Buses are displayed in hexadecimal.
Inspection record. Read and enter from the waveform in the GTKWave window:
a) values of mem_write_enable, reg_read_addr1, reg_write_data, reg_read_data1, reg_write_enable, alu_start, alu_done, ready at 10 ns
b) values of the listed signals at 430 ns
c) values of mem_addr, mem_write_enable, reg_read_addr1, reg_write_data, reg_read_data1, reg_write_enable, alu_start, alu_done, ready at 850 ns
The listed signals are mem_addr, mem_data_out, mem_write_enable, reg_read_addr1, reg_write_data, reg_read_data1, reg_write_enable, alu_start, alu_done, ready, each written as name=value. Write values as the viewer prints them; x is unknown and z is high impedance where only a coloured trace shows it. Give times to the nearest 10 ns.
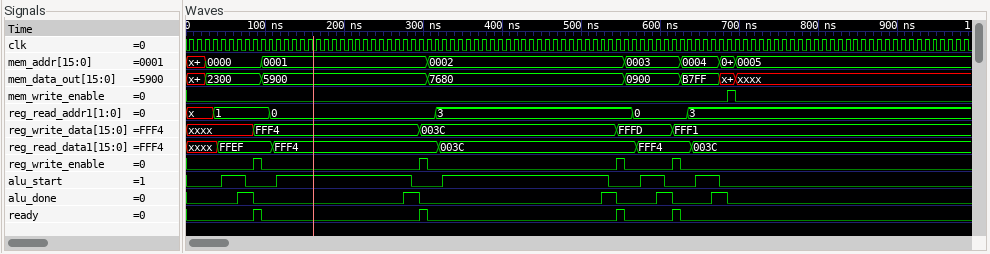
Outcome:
mem_write_enable=0, reg_read_addr1=x, reg_write_data=xxxx, reg_read_data1=xxxx, reg_write_enable=0, alu_start=0, alu_done=0, ready=0
mem_addr=0002, mem_data_out=7680, mem_write_enable=0, reg_read_addr1=3, reg_write_data=003C, reg_read_data1=003C, reg_write_enable=0, alu_start=1, alu_done=0, ready=0
mem_addr=0005, mem_write_enable=0, reg_read_addr1=3, reg_write_data=FFF1, reg_read_data1=003C, reg_write_enable=0, alu_start=0, alu_done=0, ready=0
